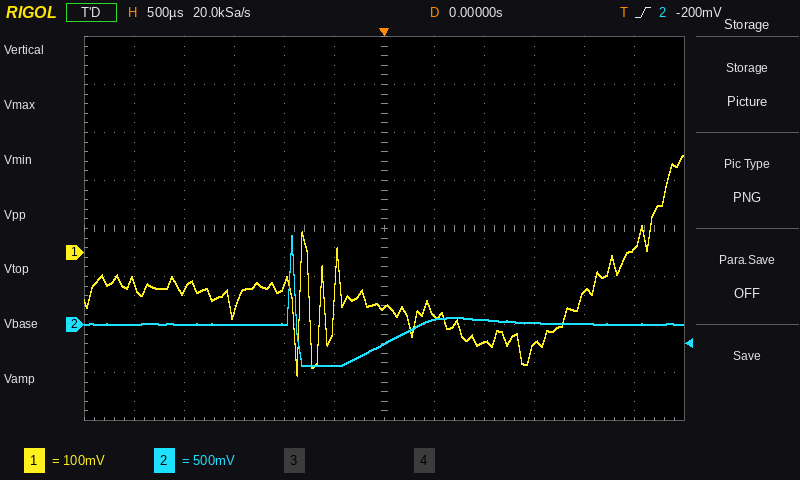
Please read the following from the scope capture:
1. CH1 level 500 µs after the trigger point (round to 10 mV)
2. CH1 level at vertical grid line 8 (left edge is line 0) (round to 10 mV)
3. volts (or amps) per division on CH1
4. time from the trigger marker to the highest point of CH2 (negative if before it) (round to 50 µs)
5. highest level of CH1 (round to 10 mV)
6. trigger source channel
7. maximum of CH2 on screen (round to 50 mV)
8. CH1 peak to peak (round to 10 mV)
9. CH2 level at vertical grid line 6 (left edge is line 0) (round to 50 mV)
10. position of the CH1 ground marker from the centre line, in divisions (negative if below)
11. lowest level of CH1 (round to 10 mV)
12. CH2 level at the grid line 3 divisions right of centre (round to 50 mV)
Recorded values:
-130 mV
-190 mV
100 mV
-900 µs
200 mV
CH2
950 mV
460 mV
-200 mV
-0.5 div
-260 mV
0 mV
